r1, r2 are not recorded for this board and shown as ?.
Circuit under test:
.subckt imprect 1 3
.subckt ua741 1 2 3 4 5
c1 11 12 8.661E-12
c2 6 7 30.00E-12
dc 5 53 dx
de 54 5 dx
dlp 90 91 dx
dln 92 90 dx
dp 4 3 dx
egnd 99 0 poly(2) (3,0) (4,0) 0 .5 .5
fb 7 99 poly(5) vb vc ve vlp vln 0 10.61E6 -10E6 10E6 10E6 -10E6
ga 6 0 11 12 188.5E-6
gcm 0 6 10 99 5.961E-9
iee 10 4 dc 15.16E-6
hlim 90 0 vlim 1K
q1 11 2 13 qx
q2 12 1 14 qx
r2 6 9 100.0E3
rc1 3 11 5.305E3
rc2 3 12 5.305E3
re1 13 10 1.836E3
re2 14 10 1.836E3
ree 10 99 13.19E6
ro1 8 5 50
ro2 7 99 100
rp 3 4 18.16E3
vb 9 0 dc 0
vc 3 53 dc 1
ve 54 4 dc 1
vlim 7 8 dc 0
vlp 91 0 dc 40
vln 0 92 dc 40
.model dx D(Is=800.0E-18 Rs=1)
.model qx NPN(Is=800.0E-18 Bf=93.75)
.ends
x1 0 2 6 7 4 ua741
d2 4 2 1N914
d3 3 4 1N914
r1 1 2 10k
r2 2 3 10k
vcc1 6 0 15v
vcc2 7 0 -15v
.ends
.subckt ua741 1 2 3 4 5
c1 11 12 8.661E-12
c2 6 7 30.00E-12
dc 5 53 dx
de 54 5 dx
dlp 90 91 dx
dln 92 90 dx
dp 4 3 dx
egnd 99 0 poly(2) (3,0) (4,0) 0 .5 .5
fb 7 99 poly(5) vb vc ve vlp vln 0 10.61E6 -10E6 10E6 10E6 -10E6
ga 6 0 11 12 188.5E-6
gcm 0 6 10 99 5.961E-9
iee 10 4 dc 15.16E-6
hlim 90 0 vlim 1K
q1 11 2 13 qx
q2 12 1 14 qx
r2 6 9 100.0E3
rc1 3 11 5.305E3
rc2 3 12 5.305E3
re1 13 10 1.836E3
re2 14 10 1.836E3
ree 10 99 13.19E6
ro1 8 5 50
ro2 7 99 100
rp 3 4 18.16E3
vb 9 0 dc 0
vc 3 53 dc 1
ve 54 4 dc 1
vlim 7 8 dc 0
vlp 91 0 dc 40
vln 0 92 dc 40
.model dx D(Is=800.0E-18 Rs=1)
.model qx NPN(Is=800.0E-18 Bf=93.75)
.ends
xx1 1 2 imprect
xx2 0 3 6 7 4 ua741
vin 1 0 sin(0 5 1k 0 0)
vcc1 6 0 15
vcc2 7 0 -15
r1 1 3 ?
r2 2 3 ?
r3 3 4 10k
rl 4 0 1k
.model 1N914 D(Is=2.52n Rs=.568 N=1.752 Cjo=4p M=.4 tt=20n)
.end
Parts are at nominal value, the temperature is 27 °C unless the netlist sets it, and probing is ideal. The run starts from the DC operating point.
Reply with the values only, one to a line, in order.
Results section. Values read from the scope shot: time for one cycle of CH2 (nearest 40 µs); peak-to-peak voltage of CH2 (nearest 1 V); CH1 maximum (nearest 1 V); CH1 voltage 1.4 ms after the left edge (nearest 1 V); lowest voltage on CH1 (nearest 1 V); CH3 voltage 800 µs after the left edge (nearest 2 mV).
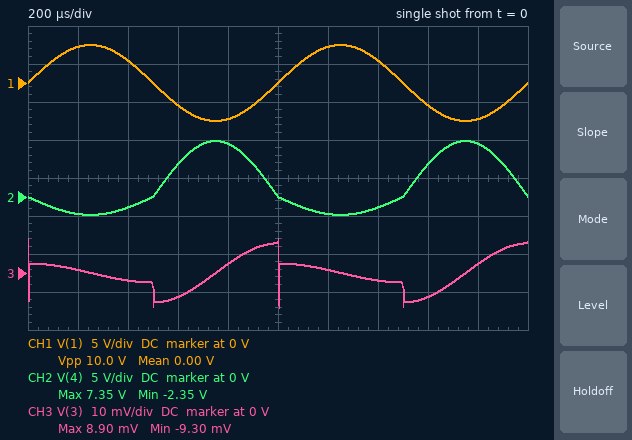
1.00 ms
10 V
5 V
3 V
-5 V
2 mV
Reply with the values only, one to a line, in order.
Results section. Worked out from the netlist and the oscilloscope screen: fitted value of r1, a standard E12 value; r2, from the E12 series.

6.8 kΩ
10 kΩ
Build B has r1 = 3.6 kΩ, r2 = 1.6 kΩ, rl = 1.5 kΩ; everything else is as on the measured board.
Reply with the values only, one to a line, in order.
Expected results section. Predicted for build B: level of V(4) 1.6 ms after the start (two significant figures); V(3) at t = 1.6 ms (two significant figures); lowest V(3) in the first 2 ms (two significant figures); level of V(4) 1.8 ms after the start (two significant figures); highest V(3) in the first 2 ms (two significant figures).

8.1 V
-12 mV
-270 mV
13 V
18 mV
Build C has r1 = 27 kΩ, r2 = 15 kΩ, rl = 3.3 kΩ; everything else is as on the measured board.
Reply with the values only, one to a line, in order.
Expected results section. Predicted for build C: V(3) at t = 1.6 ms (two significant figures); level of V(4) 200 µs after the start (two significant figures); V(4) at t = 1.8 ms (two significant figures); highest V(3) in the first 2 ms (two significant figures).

-1.5 mV
1.4 V
1.8 V
2.8 mV
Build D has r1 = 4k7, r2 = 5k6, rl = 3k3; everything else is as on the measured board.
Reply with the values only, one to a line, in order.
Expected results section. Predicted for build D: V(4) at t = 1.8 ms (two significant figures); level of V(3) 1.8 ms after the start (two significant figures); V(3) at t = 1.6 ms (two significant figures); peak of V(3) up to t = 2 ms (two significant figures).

10 V
3.3 mV
-8.9 mV
12 mV
